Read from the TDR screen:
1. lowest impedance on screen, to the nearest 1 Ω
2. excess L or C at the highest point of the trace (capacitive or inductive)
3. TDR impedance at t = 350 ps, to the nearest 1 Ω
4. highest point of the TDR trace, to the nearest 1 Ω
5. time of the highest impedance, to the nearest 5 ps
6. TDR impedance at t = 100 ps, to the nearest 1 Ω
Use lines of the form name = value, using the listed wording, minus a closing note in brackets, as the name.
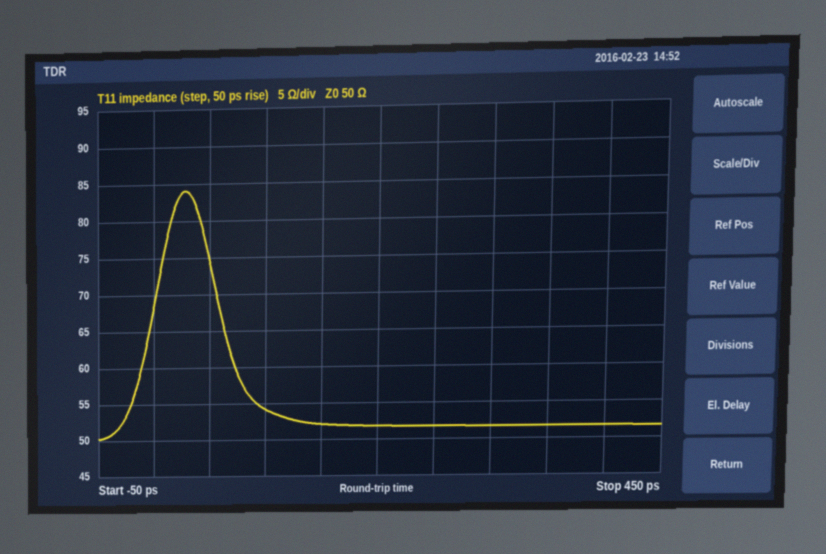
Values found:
lowest impedance on screen, to the nearest 1 Ω = 50 Ω
excess L or C at the highest point of the trace = inductive
TDR impedance at t = 350 ps, to the nearest 1 Ω = 52 Ω
highest point of the TDR trace, to the nearest 1 Ω = 84 Ω
time of the highest impedance, to the nearest 5 ps = 30 ps
TDR impedance at t = 100 ps, to the nearest 1 Ω = 54 Ω
